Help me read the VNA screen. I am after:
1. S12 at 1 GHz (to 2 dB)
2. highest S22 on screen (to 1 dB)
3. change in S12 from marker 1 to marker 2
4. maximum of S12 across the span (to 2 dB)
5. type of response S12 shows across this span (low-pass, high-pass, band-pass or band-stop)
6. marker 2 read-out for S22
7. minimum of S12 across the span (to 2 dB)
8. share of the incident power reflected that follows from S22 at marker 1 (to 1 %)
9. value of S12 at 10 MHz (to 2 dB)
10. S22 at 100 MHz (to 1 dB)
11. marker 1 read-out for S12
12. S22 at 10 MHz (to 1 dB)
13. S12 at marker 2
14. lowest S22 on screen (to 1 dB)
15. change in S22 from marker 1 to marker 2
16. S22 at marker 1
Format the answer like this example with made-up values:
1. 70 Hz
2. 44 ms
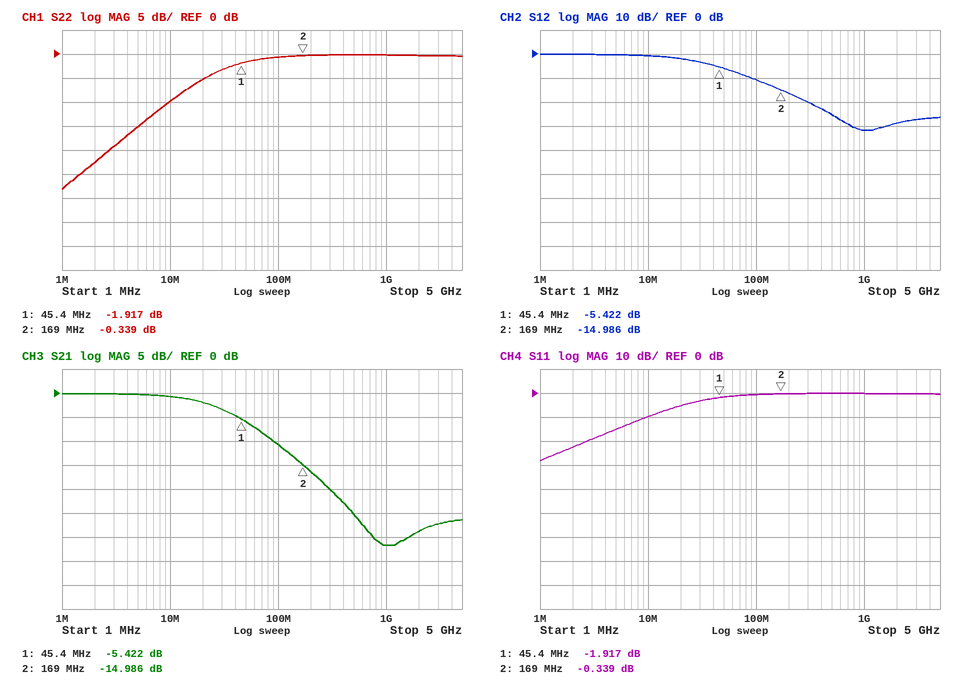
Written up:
1. -32 dB
2. 0 dB
3. -9.564 dB
4. 0 dB
5. low-pass
6. -0.339 dB
7. -32 dB
8. 64 %
9. 0 dB
10. -1 dB
11. -5.422 dB
12. -10 dB
13. -14.986 dB
14. -28 dB
15. 1.578 dB
16. -1.917 dB
